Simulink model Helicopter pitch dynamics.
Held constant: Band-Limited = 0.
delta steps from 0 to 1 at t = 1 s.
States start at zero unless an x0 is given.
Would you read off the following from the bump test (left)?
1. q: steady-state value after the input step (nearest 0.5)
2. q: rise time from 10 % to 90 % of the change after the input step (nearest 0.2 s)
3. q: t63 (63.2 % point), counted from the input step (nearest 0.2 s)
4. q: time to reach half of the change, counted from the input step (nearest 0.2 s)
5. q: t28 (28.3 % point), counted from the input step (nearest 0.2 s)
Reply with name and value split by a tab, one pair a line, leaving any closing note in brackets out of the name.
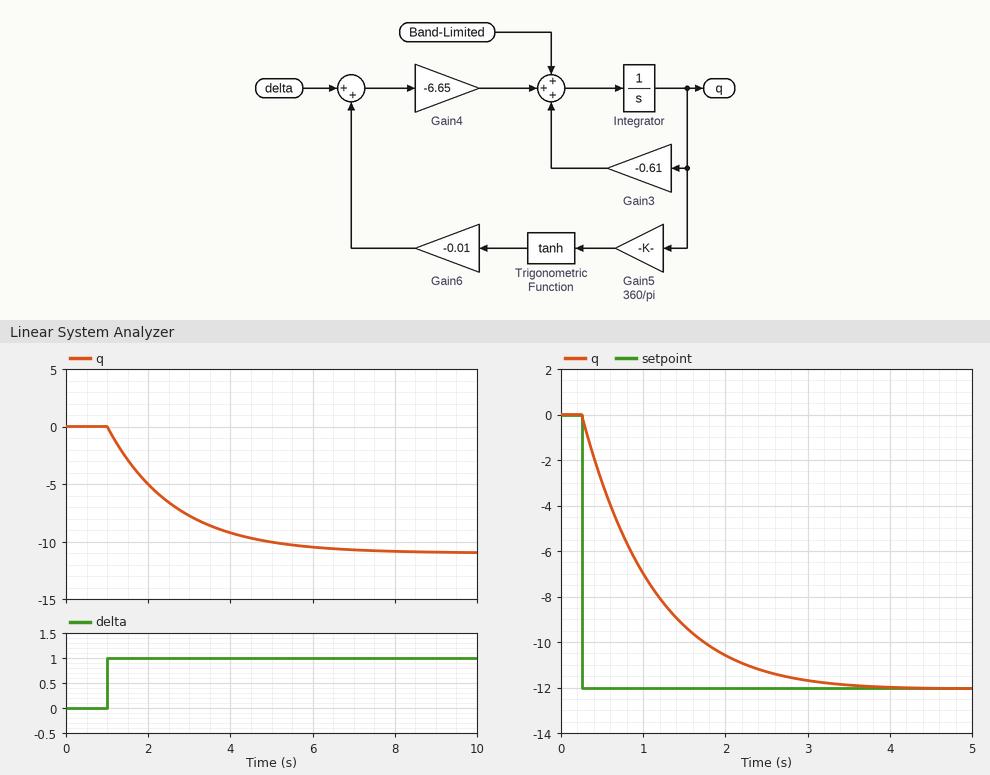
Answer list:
q: steady-state value after the input step	-11.0
q: rise time from 10 % to 90 % of the change after the input step	3.6 s
q: t63 (63.2 % point), counted from the input step	1.6 s
q: time to reach half of the change, counted from the input step	1.2 s
q: t28 (28.3 % point), counted from the input step	0.6 s
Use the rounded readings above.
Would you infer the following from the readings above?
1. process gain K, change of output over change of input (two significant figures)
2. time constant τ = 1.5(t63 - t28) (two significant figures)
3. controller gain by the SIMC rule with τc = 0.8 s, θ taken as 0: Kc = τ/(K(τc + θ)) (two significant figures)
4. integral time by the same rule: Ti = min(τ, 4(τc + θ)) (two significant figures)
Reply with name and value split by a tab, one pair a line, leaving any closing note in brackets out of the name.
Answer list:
process gain K, change of output over change of input	-11
time constant τ = 1.5(t63 - t28)	1.5 s
controller gain by the SIMC rule with τc = 0.8 s, θ taken as 0: Kc = τ/(K(τc + θ))	-0.17
integral time by the same rule: Ti = min(τ, 4(τc + θ))	1.5 s
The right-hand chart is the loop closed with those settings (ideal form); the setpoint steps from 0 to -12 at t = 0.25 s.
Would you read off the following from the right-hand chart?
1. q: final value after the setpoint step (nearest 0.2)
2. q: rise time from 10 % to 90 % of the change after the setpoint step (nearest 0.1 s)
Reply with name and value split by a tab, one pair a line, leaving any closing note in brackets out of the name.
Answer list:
q: final value after the setpoint step	-12.0
q: rise time from 10 % to 90 % of the change after the setpoint step	1.8 s
